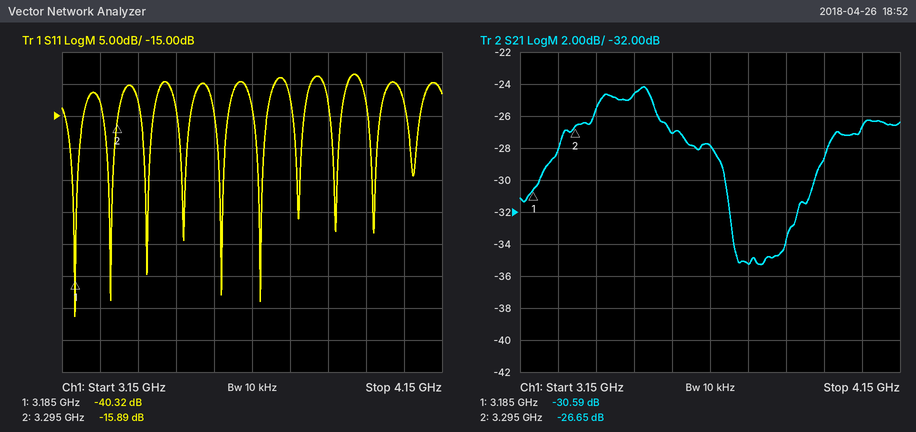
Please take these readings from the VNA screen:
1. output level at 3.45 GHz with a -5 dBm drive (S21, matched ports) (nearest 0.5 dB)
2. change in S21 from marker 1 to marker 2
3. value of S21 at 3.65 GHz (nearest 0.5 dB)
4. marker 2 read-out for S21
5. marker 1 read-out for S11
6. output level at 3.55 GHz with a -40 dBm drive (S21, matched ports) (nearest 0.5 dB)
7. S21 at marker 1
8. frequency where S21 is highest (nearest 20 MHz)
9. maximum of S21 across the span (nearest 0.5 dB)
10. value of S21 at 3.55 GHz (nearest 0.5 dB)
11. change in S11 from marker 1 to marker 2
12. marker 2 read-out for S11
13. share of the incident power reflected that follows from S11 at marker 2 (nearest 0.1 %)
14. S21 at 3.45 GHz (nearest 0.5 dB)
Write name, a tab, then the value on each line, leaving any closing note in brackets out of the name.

output level at 3.45 GHz with a -5 dBm drive (S21, matched ports)	-29.5 dBm
change in S21 from marker 1 to marker 2	3.94 dB
value of S21 at 3.65 GHz	-28.0 dB
marker 2 read-out for S21	-26.65 dB
marker 1 read-out for S11	-40.32 dB
output level at 3.55 GHz with a -40 dBm drive (S21, matched ports)	-67.0 dBm
S21 at marker 1	-30.59 dB
frequency where S21 is highest	3.48 GHz
maximum of S21 across the span	-24.0 dB
value of S21 at 3.55 GHz	-27.0 dB
change in S11 from marker 1 to marker 2	24.43 dB
marker 2 read-out for S11	-15.89 dB
share of the incident power reflected that follows from S11 at marker 2	2.6 %
S21 at 3.45 GHz	-24.5 dB
